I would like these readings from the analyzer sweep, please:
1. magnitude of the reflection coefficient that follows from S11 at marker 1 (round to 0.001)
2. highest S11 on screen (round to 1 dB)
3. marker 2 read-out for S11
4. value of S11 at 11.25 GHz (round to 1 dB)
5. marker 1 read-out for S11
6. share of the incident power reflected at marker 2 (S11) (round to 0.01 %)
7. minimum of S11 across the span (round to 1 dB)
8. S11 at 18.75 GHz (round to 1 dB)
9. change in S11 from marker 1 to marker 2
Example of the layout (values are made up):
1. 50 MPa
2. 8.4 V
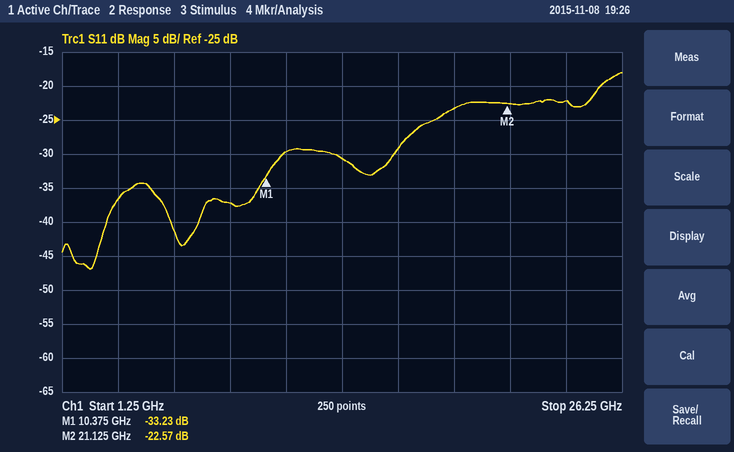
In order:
1. 0.022
2. -18 dB
3. -22.57 dB
4. -30 dB
5. -33.23 dB
6. 0.55 %
7. -47 dB
8. -23 dB
9. 10.66 dB
